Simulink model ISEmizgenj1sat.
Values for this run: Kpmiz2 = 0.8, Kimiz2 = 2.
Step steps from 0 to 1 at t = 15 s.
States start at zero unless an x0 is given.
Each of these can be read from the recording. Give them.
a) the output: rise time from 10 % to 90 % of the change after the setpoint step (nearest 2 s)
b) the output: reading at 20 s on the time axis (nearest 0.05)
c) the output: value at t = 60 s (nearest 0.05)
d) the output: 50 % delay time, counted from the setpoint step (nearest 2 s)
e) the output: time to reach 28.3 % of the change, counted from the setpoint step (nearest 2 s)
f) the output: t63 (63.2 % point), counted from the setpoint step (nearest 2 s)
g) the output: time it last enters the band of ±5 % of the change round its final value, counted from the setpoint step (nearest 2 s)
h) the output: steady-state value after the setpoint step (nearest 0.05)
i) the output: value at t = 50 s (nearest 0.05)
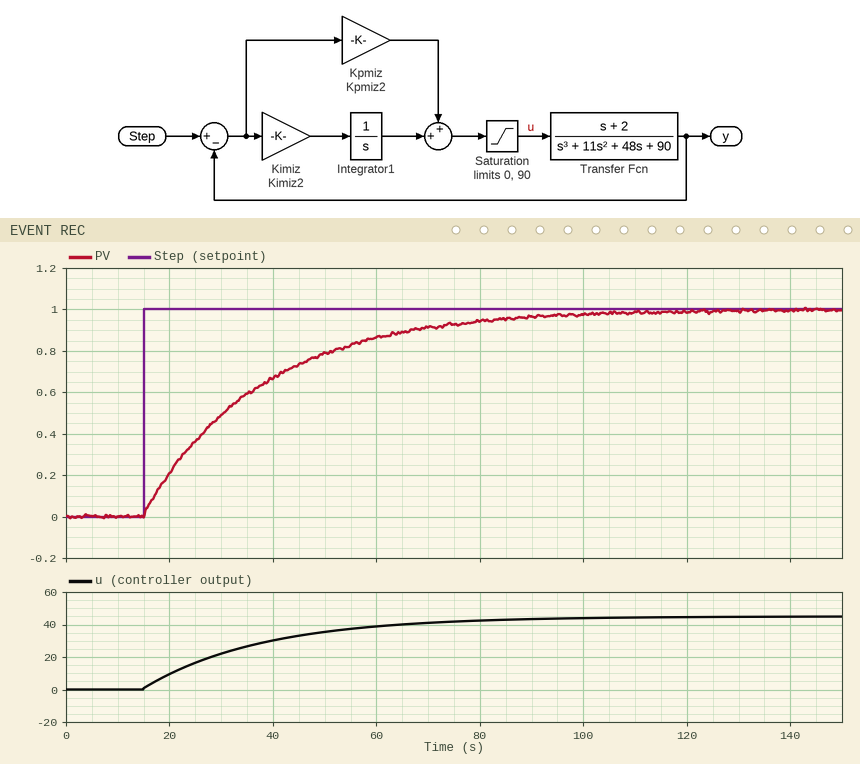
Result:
50 s
0.20
0.85
16 s
8 s
22 s
68 s
1.00
0.80
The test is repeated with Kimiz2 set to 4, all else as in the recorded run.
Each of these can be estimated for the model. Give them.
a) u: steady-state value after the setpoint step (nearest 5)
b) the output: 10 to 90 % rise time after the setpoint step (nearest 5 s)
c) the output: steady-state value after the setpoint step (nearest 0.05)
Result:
45
25 s
1.00
